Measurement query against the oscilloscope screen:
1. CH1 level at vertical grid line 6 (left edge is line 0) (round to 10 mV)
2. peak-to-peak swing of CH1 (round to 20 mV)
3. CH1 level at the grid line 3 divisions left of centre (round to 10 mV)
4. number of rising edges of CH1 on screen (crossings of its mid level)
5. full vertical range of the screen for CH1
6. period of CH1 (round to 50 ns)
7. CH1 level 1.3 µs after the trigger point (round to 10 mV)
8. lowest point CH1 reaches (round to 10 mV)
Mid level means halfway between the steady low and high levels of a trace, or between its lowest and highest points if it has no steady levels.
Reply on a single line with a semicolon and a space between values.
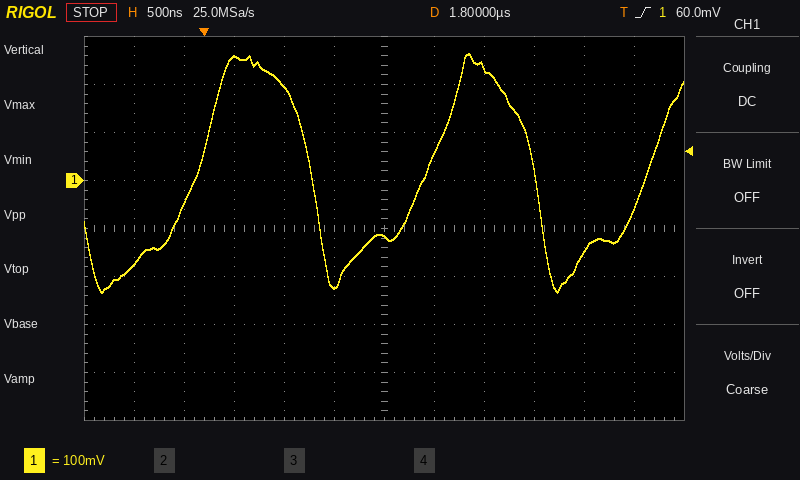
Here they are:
-120 mV; 500 mV; 260 mV; 3; 800 mV; 2.25 µs; -220 mV; -230 mV
